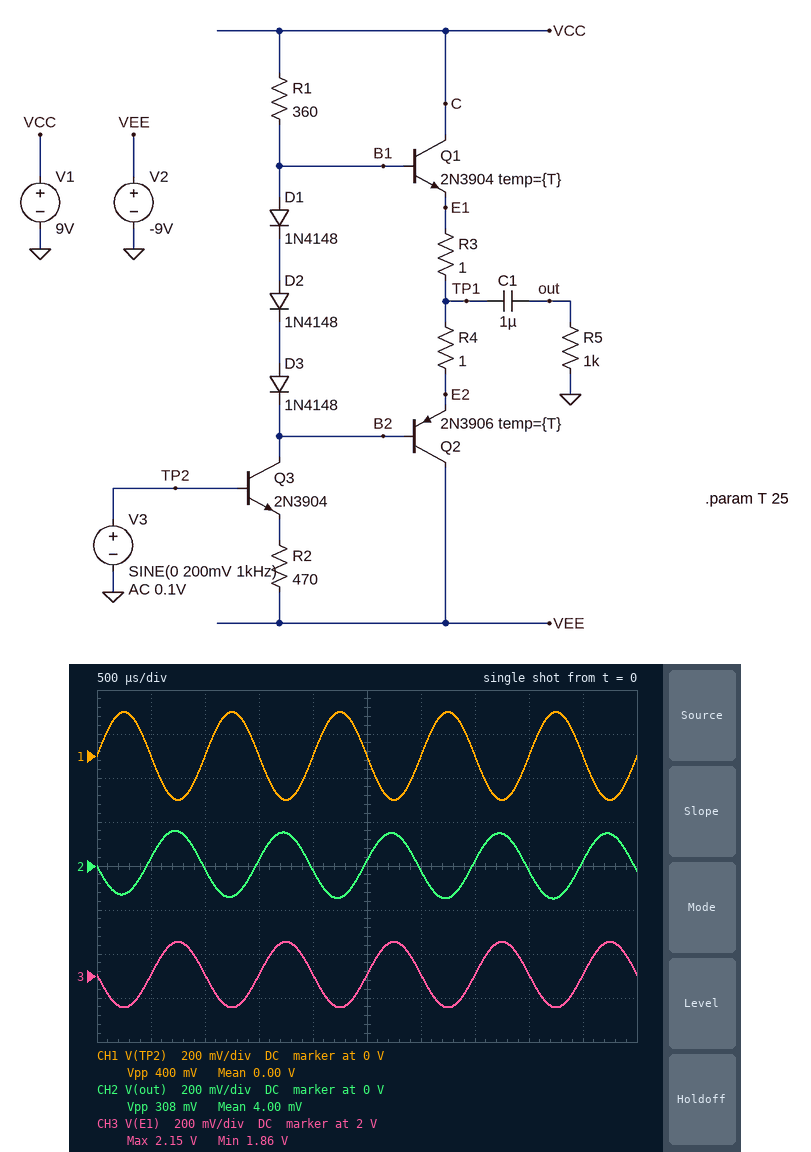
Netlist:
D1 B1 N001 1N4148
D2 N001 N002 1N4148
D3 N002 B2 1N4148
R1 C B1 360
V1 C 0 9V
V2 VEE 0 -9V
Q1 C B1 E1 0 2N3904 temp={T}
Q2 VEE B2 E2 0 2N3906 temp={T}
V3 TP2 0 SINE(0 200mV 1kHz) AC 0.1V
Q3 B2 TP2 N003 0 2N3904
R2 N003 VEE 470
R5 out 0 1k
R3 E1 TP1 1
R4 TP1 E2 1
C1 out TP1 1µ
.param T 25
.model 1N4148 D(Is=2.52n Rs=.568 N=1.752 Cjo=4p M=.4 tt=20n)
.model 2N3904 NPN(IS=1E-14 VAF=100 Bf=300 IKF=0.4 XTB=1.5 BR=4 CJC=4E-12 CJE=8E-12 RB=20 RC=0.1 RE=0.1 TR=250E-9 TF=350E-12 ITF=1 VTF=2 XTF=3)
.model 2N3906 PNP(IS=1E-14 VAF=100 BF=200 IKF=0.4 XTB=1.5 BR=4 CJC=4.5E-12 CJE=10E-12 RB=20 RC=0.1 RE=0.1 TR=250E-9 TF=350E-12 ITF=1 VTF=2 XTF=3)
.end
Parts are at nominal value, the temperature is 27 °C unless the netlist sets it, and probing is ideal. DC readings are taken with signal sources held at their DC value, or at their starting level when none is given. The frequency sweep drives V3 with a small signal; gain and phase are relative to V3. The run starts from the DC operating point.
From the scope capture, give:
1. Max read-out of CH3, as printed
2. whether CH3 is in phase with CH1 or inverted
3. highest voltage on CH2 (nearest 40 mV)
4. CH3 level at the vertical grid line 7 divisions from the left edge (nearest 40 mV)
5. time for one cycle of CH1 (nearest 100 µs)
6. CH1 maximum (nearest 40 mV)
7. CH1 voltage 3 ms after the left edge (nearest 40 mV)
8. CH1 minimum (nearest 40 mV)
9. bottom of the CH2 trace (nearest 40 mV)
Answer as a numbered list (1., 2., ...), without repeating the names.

1. 2.15 V
2. inverted
3. 160 mV
4. 2.00 V
5. 1.0 ms
6. 200 mV
7. 0 V
8. -200 mV
9. -160 mV
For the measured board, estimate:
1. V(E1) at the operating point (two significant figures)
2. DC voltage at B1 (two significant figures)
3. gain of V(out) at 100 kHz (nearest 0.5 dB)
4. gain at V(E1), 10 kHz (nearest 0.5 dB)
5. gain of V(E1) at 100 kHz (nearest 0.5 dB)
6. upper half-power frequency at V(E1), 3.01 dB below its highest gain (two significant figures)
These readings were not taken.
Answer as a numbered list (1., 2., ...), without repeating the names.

1. 2.0 V
2. 2.9 V
3. -2.5 dB
4. -2.5 dB
5. -2.5 dB
6. 99 MHz
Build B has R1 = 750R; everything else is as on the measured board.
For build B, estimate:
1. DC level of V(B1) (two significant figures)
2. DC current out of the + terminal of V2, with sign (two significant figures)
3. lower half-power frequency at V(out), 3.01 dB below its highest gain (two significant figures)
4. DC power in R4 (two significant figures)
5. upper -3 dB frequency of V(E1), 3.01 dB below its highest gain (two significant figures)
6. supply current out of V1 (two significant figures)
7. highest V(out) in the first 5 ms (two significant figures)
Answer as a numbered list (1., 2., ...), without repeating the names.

1. 1.2 V
2. -210 mA
3. 170 Hz
4. 38 mW
5. 1.3 GHz
6. 200 mA
7. 180 mV
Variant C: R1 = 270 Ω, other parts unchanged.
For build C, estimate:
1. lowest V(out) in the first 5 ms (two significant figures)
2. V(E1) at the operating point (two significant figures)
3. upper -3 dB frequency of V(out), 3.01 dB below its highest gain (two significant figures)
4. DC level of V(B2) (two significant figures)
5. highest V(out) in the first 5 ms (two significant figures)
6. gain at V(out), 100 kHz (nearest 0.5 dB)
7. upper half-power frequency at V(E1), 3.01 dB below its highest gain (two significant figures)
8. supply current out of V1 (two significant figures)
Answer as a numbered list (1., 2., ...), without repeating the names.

1. -110 mV
2. 3.5 V
3. 180 MHz
4. 2.2 V
5. 120 mV
6. -5.0 dB
7. 190 MHz
8. 240 mA
